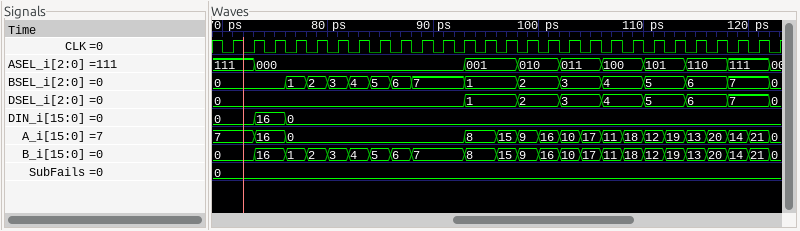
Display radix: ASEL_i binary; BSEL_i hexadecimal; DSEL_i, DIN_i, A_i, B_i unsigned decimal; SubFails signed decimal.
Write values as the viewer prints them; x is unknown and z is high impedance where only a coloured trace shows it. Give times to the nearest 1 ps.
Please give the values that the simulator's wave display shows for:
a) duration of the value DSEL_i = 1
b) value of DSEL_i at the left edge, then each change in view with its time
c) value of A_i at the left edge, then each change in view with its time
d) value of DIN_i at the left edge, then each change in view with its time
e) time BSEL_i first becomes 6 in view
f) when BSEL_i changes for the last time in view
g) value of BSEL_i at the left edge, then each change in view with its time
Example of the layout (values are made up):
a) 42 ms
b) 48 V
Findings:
a) 5 ps
b) 0, 1 at 93 ps, 2 at 98 ps, 3 at 102 ps, 4 at 106 ps, 5 at 110 ps, 6 at 114 ps, 7 at 118 ps, 0 at 122 ps
c) 7, 16 at 73 ps, 0 at 76 ps, 8 at 93 ps, 15 at 96 ps, 9 at 98 ps, 16 at 100 ps, 10 at 102 ps, 17 at 104 ps, 11 at 106 ps, 18 at 108 ps, 12 at 110 ps, 19 at 112 ps, 13 at 114 ps, 20 at 116 ps, 14 at 118 ps, 21 at 120 ps, 0 at 122 ps
d) 0, 16 at 73 ps, 0 at 76 ps
e) 86 ps
f) 122 ps
g) 0, 1 at 76 ps, 2 at 78 ps, 3 at 80 ps, 4 at 82 ps, 5 at 84 ps, 6 at 86 ps, 7 at 88 ps, 1 at 93 ps, 2 at 98 ps, 3 at 102 ps, 4 at 106 ps, 5 at 110 ps, 6 at 114 ps, 7 at 118 ps, 0 at 122 ps
